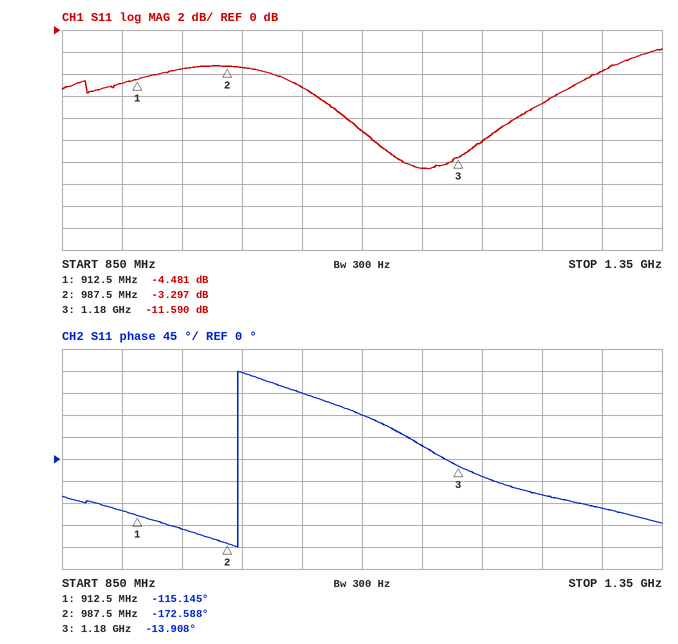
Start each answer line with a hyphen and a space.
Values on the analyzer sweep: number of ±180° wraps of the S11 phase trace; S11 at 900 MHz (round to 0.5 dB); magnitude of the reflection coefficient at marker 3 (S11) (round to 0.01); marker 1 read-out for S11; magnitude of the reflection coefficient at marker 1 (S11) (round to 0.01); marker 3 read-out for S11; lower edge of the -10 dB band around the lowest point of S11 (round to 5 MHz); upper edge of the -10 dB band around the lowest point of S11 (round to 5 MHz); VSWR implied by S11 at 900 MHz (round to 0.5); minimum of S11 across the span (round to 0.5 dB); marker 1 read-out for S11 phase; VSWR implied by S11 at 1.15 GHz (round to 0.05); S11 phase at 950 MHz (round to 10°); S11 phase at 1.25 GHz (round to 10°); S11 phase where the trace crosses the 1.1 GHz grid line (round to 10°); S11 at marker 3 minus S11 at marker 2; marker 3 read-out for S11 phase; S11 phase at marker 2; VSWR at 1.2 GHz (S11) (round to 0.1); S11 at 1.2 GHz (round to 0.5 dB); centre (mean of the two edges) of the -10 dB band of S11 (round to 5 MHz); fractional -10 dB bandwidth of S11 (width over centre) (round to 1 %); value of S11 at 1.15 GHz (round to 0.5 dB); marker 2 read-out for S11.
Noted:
- 1
- -5.0 dB
- 0.26
- -4.481 dB
- 0.60
- -11.590 dB
- 1.110 GHz
- 1.200 GHz
- 3.5
- -12.5 dB
- -115.145°
- 1.60
- -140°
- -70°
- 90°
- -8.293 dB
- -13.908°
- -172.588°
- 1.9
- -10.0 dB
- 1.155 GHz
- 8 %
- -12.5 dB
- -3.297 dB
